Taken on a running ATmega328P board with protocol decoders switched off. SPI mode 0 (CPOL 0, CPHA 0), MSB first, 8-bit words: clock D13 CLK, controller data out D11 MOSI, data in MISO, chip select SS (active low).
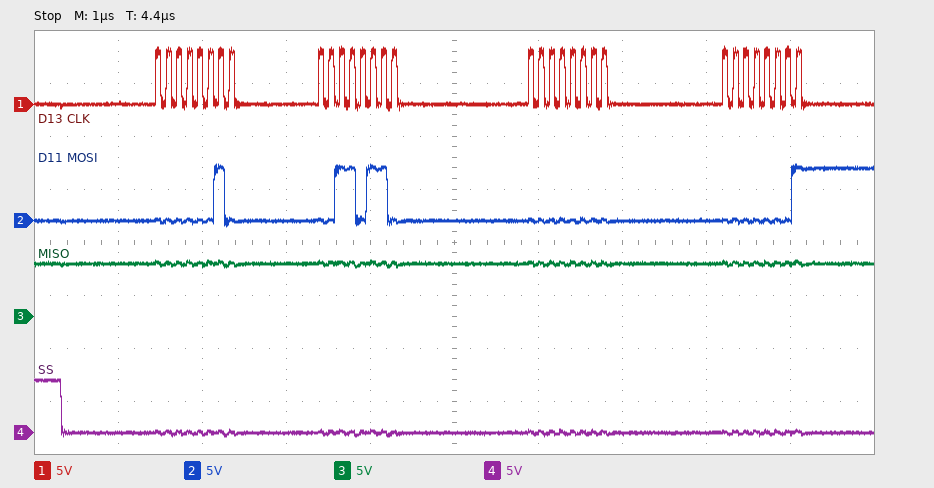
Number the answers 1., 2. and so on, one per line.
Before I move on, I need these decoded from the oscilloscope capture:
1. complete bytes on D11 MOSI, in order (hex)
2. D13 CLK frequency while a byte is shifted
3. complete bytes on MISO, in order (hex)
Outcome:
1. 02 36 00 01
2. 8 MHz
3. FF FF FF FF
